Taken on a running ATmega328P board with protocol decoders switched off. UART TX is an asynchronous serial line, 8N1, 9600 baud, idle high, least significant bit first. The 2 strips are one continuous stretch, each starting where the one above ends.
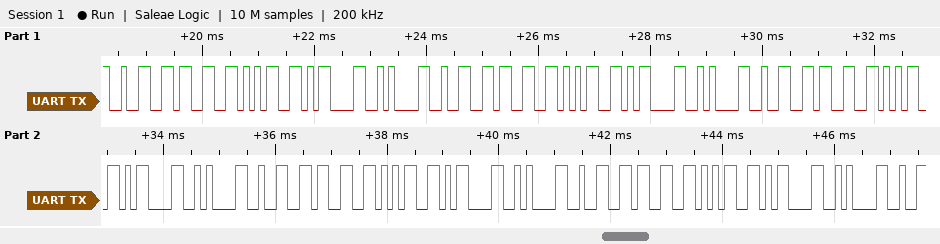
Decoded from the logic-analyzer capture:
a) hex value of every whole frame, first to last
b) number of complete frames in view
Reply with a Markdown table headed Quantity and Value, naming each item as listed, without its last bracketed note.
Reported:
| Quantity | Value |
|---|---|
| hex value of every whole frame, first to last | 32 33 35 0D 0A 32 33 35 0D 0A 32 33 35 0D 0A 32 33 35 0D 0A 32 33 35 0D 0A |
| number of complete frames in view | 25 |
